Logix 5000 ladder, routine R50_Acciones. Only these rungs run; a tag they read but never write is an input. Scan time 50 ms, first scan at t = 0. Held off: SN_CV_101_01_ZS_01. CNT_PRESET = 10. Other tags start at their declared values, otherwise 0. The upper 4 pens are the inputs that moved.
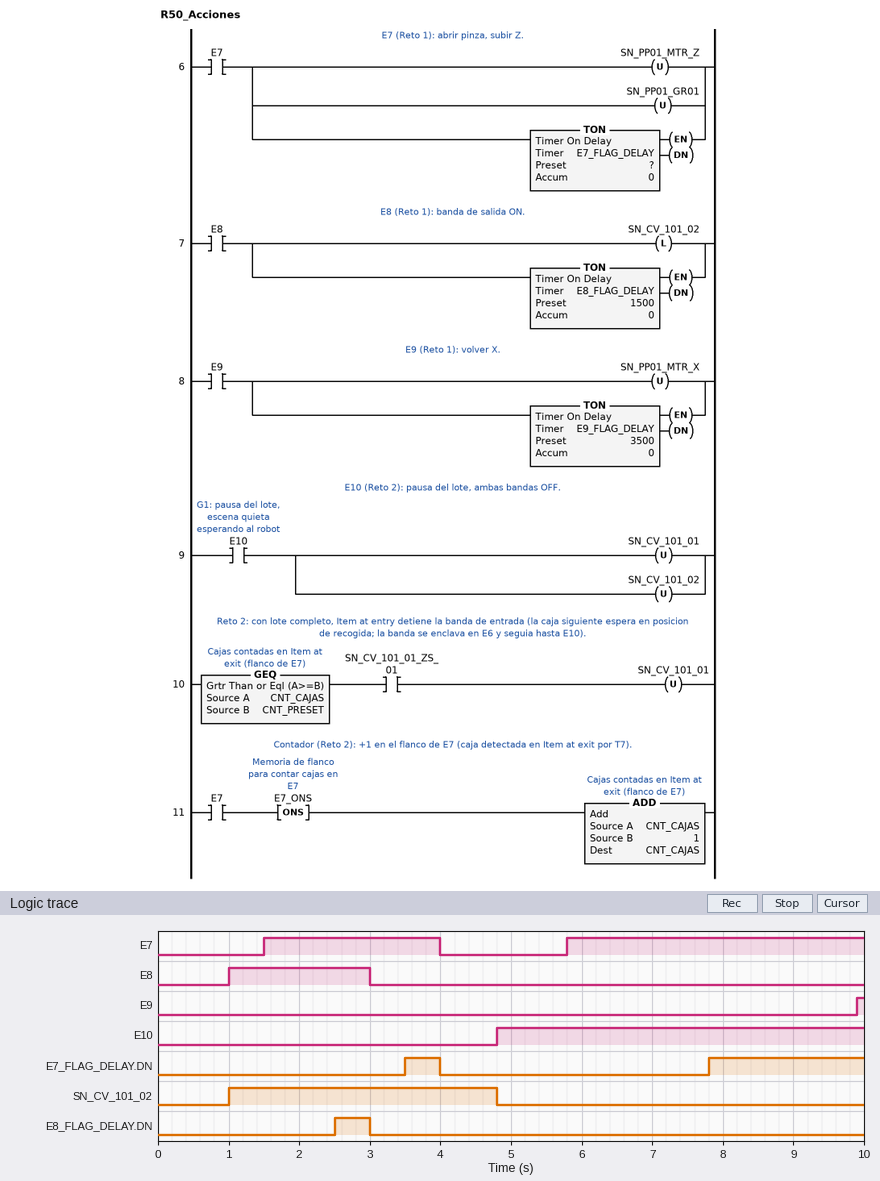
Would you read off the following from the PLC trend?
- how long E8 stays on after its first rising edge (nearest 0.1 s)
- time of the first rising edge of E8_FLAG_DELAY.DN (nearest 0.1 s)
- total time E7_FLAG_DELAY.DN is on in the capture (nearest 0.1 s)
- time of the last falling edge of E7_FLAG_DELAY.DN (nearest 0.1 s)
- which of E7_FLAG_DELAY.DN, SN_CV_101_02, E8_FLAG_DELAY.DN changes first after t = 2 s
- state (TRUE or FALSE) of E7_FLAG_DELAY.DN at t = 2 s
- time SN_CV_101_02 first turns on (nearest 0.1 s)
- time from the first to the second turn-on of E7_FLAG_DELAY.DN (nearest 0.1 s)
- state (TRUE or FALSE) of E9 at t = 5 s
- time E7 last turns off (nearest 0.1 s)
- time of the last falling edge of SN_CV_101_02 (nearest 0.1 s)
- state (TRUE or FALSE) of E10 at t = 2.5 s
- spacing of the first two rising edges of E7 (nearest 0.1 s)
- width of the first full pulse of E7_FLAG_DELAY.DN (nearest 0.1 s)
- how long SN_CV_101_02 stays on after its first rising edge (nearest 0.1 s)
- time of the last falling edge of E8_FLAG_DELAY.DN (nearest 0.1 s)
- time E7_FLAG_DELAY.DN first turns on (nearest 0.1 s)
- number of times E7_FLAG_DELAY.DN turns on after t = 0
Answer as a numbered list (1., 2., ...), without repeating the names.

1. 2.0 s
2. 2.5 s
3. 2.7 s
4. 4.0 s
5. E8_FLAG_DELAY.DN
6. FALSE
7. 1.0 s
8. 4.3 s
9. FALSE
10. 4.0 s
11. 4.8 s
12. FALSE
13. 4.3 s
14. 0.5 s
15. 3.8 s
16. 3.0 s
17. 3.5 s
18. 2
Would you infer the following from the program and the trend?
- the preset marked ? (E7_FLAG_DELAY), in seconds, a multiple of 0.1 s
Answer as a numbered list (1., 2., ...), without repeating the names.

1. 2.0 s
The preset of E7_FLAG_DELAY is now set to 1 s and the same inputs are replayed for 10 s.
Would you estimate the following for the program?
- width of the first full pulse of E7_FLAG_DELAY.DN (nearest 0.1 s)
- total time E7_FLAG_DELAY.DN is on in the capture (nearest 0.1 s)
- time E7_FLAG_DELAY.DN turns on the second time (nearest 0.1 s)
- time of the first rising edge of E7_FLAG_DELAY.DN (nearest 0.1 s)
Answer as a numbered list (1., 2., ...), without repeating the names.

1. 1.5 s
2. 4.7 s
3. 6.8 s
4. 2.5 s
